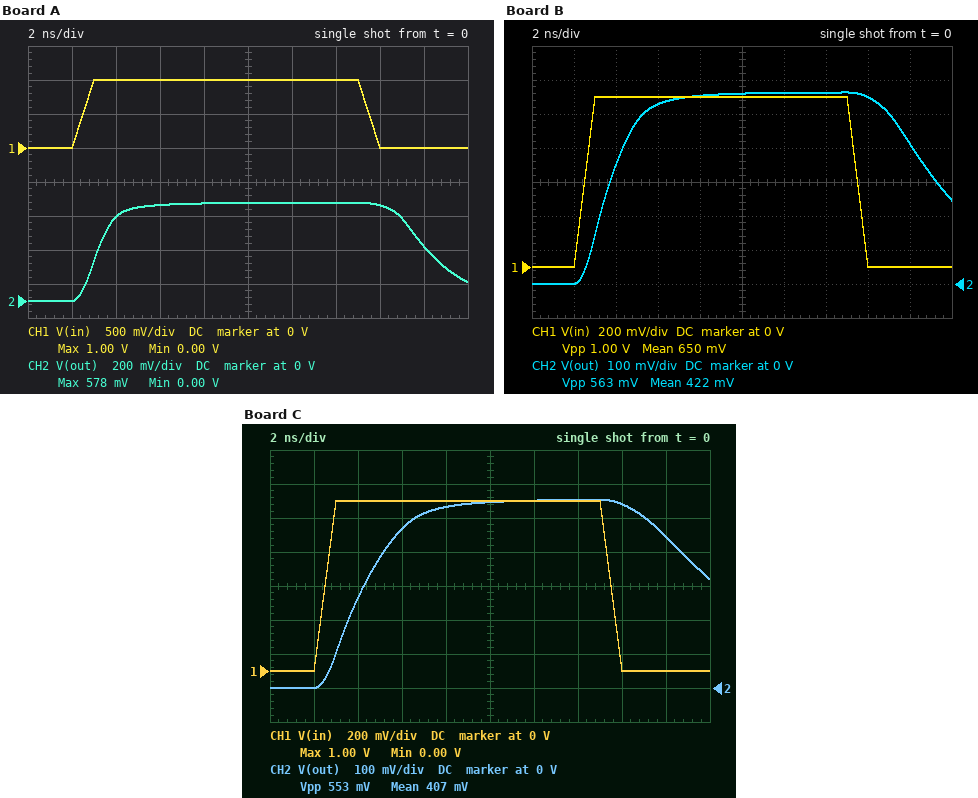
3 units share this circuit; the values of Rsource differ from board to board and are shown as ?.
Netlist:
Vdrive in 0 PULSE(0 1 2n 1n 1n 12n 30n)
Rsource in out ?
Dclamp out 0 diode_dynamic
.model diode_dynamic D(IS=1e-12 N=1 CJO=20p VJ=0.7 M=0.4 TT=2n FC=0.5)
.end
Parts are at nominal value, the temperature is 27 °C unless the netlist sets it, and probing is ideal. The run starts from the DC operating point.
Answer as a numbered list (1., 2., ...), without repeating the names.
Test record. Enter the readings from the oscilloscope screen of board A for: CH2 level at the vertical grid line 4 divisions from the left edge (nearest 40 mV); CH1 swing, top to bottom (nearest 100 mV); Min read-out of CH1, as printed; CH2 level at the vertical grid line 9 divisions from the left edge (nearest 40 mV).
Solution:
1. 560 mV
2. 1.0 V
3. 0.00 V
4. 320 mV
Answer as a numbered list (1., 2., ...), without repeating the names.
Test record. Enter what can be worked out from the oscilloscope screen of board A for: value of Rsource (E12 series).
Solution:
1. 82 Ω
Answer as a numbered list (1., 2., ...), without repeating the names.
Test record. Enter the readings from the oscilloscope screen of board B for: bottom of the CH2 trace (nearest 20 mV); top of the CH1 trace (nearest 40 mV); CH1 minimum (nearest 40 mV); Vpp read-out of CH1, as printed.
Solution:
1. 0 V
2. 1.00 V
3. 0 V
4. 1.00 V
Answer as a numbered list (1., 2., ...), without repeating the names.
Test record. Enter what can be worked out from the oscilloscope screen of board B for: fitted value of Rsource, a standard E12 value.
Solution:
1. 150 Ω
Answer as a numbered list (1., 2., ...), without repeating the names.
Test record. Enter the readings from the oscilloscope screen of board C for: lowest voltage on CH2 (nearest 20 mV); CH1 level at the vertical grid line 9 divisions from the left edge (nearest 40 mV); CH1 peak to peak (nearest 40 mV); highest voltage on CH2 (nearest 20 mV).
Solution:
1. 0 V
2. 0 V
3. 1.00 V
4. 560 mV
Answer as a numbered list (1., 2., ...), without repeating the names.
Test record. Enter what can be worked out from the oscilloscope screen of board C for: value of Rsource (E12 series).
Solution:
1. 220 Ω
